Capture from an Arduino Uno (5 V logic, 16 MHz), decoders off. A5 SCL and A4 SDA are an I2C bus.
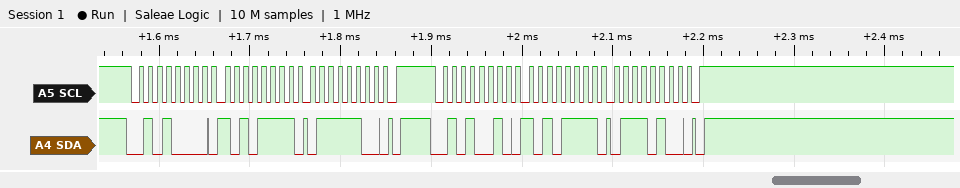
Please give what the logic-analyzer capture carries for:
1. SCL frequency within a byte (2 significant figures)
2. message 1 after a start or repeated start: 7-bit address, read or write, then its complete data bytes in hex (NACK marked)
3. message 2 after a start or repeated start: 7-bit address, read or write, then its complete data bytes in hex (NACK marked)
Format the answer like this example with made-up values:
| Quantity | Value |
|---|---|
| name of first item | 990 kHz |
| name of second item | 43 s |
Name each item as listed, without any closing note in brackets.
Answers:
| Quantity | Value |
|---|---|
| SCL frequency within a byte | 100 kHz |
| message 1 after a start or repeated start: 7-bit address, read or write, then its complete data bytes in hex | 0x28 write: AF 7C |
| message 2 after a start or repeated start: 7-bit address, read or write, then its complete data bytes in hex | 0x29 write: AF 74 |
